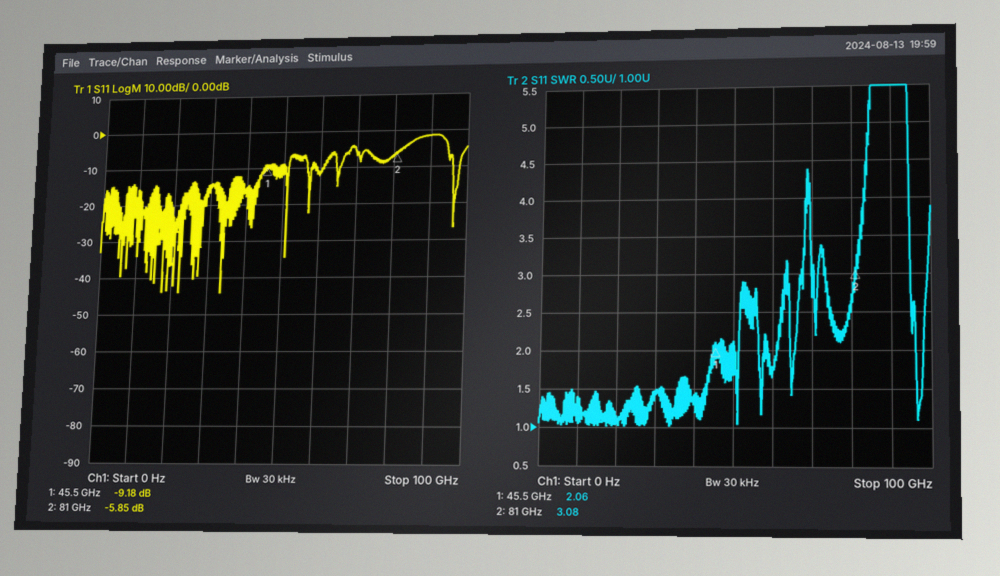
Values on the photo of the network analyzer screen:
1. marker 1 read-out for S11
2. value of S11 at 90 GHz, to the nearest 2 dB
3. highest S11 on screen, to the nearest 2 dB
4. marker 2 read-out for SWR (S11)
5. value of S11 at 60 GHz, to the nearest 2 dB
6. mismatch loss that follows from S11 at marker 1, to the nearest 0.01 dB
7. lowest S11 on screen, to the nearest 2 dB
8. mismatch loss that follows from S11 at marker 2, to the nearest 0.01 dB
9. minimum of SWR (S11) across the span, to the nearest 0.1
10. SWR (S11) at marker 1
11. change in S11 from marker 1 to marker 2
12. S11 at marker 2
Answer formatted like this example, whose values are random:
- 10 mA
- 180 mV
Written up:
- -9.18 dB
- -2 dB
- -2 dB
- 3.08
- -12 dB
- 0.56 dB
- -44 dB
- 1.31 dB
- 1.0
- 2.06
- 3.33 dB
- -5.85 dB
